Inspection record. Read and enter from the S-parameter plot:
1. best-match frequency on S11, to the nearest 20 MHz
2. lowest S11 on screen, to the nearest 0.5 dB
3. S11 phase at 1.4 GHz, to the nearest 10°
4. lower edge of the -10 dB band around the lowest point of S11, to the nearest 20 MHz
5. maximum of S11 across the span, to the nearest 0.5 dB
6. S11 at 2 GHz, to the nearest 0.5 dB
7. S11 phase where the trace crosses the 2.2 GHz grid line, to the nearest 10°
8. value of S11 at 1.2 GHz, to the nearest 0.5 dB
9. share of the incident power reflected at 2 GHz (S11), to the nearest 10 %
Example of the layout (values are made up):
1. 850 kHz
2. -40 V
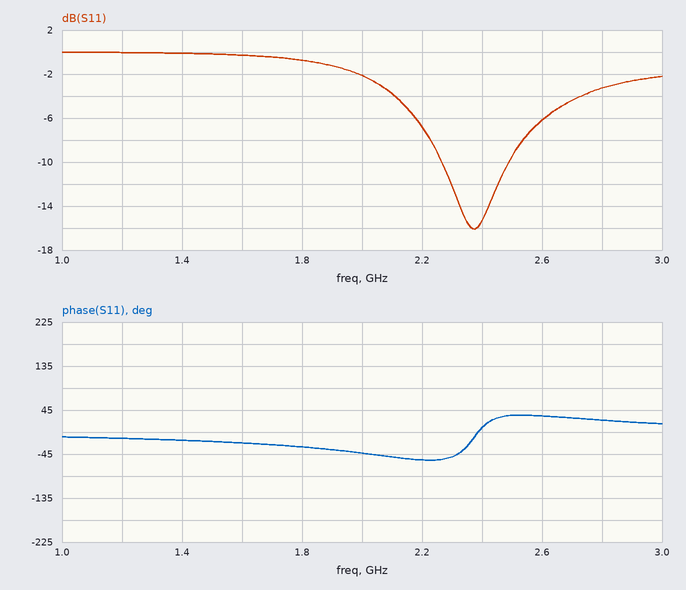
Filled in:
1. 2.38 GHz
2. -16.0 dB
3. -20°
4. 2.26 GHz
5. 0.0 dB
6. -2.0 dB
7. -60°
8. 0.0 dB
9. 60 %
